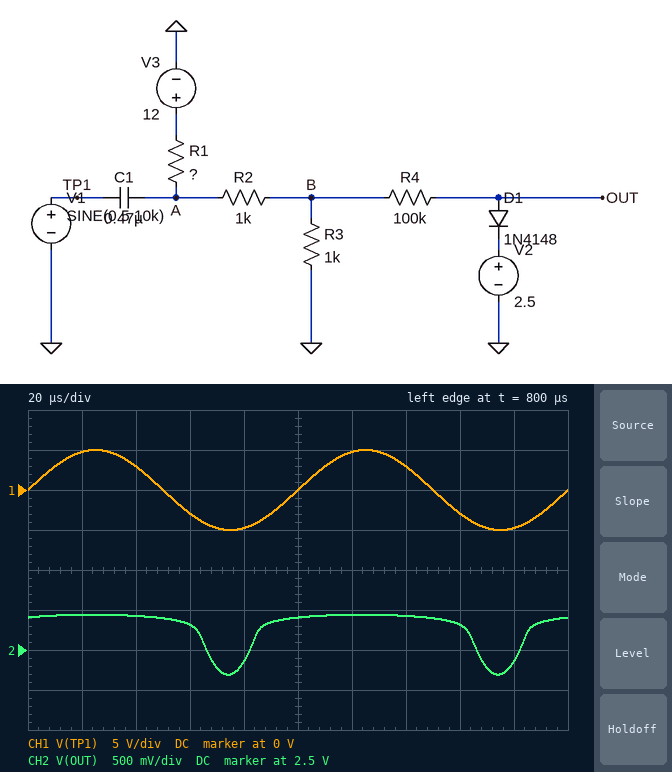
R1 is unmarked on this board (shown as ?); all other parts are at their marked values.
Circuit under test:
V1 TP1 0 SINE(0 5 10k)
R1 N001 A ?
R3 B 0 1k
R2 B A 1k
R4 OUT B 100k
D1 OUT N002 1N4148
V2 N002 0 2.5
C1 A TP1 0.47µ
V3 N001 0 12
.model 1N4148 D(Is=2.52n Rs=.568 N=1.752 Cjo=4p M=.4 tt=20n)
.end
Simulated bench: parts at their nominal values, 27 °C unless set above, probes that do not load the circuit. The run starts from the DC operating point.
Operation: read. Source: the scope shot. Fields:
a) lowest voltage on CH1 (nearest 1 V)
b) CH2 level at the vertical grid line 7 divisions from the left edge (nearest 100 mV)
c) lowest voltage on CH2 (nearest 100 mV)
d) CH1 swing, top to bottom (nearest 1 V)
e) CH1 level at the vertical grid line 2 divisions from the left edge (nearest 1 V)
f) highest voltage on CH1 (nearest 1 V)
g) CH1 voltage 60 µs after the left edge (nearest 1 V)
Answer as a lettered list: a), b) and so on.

a) -5 V
b) 2.9 V
c) 2.2 V
d) 10 V
e) 3 V
f) 5 V
g) -3 V
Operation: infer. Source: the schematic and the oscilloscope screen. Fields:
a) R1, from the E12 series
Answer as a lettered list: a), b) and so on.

a) 560 Ω
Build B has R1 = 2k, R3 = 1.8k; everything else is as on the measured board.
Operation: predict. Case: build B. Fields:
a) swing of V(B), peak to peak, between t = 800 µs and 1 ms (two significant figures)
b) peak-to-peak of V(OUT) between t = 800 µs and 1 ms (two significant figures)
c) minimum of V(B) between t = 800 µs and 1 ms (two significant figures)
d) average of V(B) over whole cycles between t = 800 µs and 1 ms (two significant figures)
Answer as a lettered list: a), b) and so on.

a) 6.4 V
b) 1.7 V
c) 1.3 V
d) 4.5 V
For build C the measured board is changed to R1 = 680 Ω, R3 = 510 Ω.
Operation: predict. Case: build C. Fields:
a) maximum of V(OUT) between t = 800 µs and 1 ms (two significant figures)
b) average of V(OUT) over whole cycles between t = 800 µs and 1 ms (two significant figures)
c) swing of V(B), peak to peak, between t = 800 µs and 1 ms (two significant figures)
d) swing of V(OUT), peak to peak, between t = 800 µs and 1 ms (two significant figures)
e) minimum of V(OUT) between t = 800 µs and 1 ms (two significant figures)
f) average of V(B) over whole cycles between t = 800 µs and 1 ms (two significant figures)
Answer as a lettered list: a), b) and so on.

a) 2.9 V
b) 2.3 V
c) 3.4 V
d) 1.8 V
e) 1.1 V
f) 2.8 V
